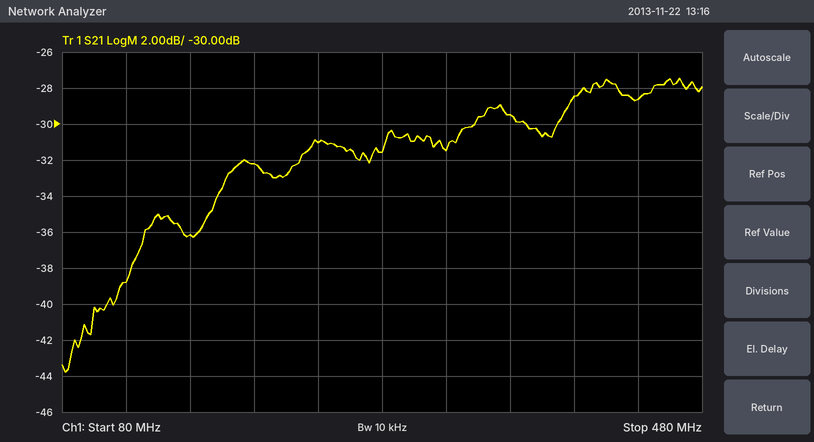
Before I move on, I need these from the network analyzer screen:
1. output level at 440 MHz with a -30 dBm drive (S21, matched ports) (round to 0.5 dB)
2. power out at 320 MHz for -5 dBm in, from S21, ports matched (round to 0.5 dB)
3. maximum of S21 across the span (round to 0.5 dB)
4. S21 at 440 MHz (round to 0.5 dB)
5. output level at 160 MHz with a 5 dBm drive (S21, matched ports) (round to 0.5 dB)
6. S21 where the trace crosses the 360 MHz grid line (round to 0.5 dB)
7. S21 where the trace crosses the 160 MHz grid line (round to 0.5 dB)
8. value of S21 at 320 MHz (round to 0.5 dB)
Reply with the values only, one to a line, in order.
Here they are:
-58.5 dBm
-36.5 dBm
-27.5 dB
-28.5 dB
-31.0 dBm
-29.5 dB
-36.0 dB
-31.5 dB
